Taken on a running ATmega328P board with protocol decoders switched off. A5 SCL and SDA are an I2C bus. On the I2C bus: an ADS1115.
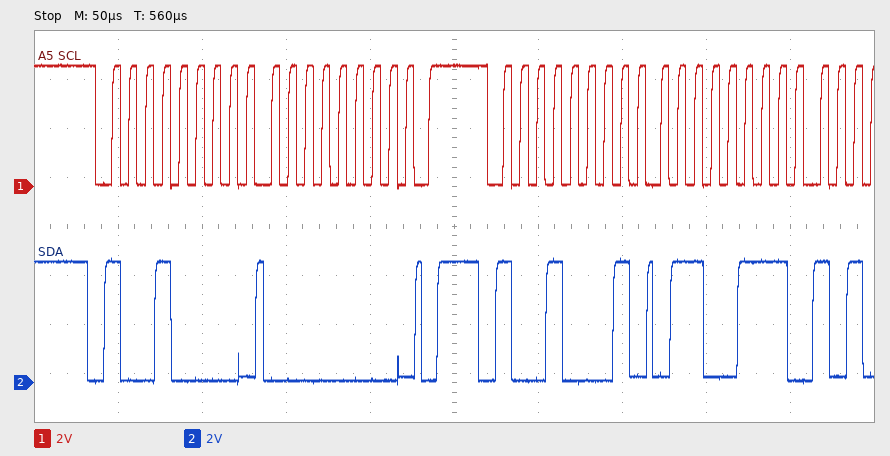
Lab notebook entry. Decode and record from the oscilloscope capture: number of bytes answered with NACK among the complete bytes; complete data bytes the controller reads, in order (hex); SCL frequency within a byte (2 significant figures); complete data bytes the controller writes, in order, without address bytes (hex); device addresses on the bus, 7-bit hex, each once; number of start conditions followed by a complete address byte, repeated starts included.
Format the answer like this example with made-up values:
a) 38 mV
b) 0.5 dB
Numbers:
a) 0
b) 67
c) 100 kHz
d) 00
e) 0x48
f) 2
